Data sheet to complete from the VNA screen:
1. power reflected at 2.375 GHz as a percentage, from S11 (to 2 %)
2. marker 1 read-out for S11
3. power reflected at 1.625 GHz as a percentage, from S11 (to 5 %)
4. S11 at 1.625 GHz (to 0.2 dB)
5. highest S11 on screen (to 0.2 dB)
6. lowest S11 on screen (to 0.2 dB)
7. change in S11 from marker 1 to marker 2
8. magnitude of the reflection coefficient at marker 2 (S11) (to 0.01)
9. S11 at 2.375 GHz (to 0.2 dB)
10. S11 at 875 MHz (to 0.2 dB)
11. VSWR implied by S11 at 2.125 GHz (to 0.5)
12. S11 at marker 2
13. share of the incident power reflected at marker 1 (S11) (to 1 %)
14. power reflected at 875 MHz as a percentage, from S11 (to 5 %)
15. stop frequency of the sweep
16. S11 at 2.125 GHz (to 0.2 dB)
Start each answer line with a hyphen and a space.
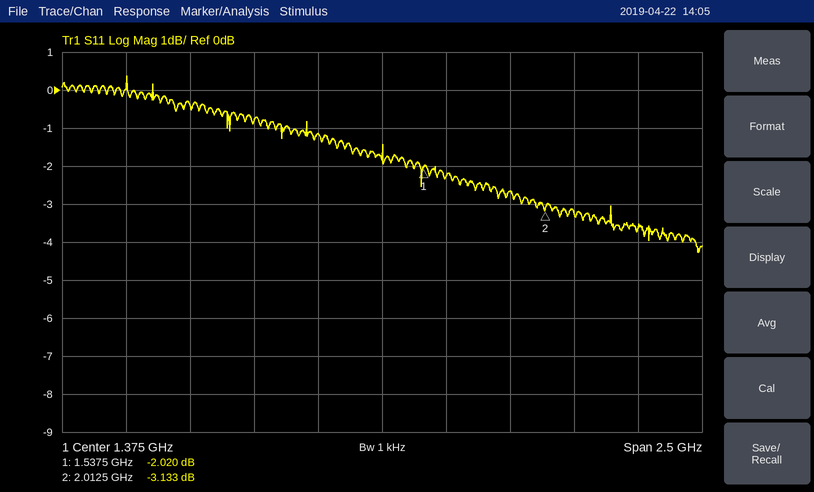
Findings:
- 44 %
- -2.020 dB
- 60 %
- -2.2 dB
- 0.4 dB
- -4.2 dB
- -1.113 dB
- 0.70
- -3.6 dB
- -0.8 dB
- 5.5
- -3.133 dB
- 63 %
- 85 %
- 2.625 GHz
- -3.2 dB
